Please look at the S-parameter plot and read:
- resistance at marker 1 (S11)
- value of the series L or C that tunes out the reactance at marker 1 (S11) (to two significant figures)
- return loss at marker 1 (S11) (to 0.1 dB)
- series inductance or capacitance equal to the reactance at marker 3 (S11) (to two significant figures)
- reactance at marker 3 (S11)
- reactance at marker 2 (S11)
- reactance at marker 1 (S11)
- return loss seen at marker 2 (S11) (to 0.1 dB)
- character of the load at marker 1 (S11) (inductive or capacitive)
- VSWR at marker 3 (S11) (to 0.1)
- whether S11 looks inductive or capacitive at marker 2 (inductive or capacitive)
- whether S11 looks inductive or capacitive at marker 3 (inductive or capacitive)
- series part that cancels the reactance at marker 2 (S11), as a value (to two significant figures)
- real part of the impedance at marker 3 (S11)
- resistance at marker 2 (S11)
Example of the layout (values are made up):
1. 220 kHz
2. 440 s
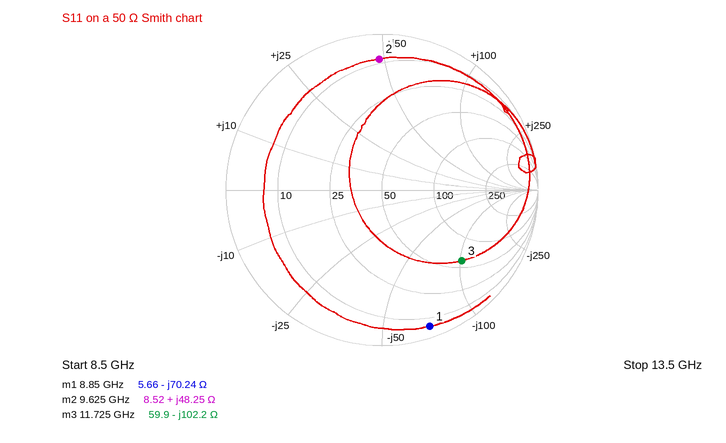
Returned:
1. 5.66 Ω
2. 1.3 nH
3. 0.7 dB
4. 130 fF
5. -102.2 Ω
6. +48.25 Ω
7. -70.24 Ω
8. 1.5 dB
9. capacitive
10. 5.3
11. inductive
12. capacitive
13. 340 fF
14. 59.9 Ω
15. 8.52 Ω
